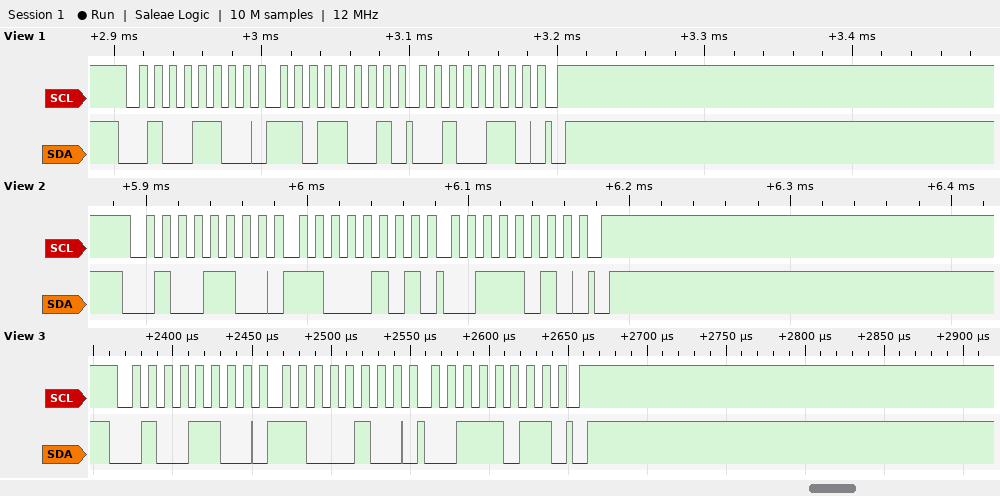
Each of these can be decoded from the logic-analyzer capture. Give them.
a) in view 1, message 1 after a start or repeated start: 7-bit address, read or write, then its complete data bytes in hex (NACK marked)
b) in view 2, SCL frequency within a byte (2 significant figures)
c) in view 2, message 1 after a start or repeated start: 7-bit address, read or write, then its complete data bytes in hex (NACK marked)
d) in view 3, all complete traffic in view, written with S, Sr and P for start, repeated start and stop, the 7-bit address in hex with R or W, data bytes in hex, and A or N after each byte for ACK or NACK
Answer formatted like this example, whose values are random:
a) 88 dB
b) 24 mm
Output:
a) 0x26 write: D9 26
b) 100 kHz
c) 0x26 write: C5 3A
d) S 26W A C4 A 3B A P
